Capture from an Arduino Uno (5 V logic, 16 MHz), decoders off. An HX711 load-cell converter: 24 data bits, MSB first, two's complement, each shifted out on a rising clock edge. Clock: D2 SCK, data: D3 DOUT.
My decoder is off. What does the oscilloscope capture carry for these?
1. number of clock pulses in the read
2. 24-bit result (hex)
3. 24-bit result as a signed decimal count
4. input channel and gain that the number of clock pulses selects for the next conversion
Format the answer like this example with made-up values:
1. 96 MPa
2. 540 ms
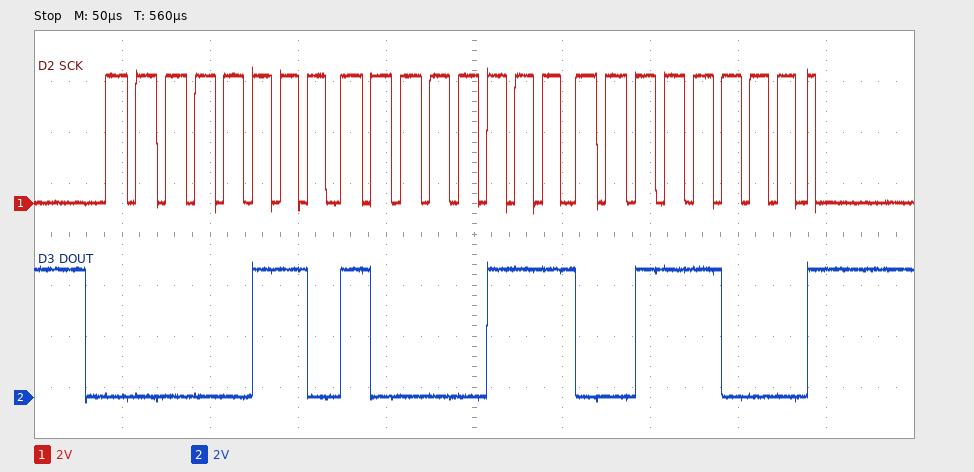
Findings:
1. 25
2. 0x068738
3. 427832
4. channel A, gain 128
